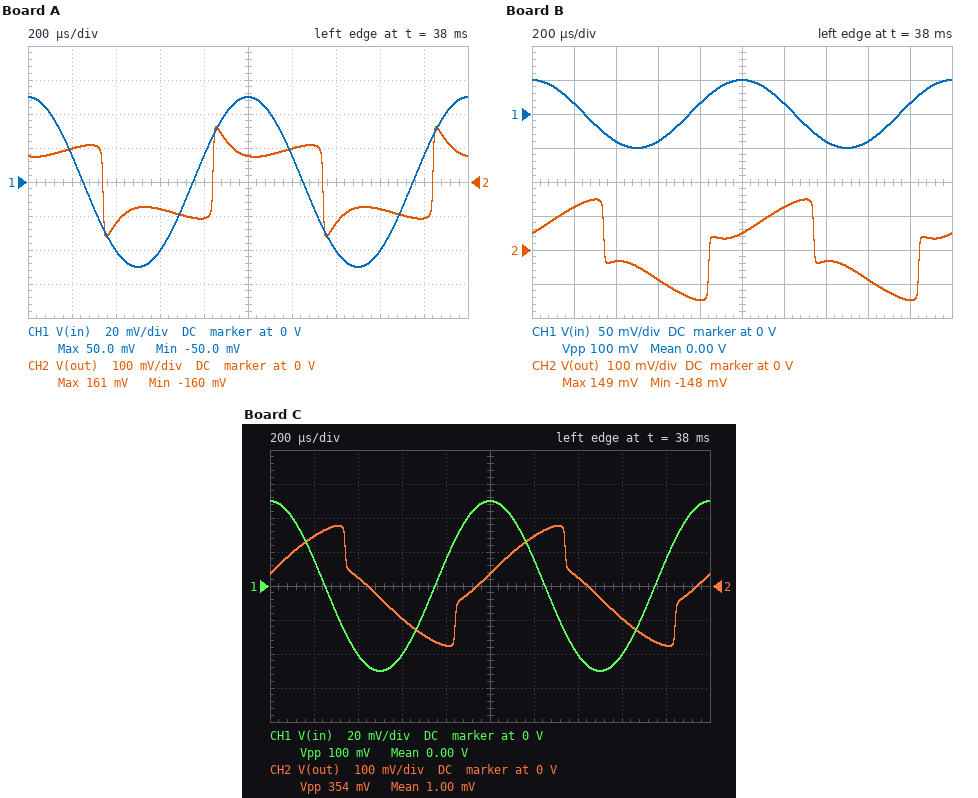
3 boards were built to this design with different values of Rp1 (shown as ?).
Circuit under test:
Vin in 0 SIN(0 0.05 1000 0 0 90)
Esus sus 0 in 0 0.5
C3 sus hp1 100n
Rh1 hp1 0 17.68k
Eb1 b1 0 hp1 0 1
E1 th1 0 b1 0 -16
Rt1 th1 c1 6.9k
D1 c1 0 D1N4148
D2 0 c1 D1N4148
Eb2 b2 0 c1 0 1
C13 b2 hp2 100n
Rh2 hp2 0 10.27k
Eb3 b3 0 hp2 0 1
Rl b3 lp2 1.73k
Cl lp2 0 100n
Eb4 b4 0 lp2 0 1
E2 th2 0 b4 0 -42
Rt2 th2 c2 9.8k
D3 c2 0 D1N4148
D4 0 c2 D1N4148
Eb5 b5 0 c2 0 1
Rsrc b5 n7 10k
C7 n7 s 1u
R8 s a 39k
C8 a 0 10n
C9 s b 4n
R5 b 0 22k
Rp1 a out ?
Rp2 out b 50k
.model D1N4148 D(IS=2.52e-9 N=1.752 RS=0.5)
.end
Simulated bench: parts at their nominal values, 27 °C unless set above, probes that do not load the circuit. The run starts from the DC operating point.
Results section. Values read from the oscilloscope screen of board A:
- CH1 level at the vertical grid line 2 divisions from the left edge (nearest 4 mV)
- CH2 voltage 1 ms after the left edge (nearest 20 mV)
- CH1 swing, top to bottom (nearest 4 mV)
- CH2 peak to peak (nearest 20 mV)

-40 mV
80 mV
100 mV
320 mV
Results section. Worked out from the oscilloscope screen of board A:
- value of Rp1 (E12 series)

68 kΩ
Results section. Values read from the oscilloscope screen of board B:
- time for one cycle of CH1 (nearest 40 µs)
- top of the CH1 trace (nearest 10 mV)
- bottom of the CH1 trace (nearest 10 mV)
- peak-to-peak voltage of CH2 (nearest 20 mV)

1.00 ms
50 mV
-50 mV
300 mV
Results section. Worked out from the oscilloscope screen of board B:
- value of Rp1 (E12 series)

33 kΩ
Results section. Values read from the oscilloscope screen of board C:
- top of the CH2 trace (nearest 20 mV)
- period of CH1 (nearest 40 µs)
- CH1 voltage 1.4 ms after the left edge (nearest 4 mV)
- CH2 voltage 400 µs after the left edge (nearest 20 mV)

180 mV
1.00 ms
-40 mV
20 mV
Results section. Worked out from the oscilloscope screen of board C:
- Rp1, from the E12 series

18 kΩ
